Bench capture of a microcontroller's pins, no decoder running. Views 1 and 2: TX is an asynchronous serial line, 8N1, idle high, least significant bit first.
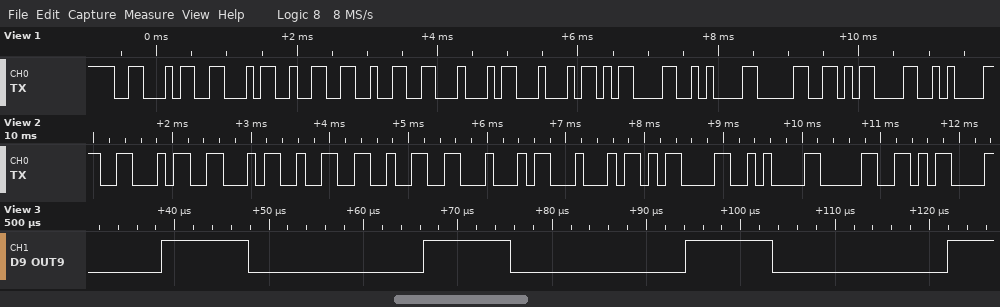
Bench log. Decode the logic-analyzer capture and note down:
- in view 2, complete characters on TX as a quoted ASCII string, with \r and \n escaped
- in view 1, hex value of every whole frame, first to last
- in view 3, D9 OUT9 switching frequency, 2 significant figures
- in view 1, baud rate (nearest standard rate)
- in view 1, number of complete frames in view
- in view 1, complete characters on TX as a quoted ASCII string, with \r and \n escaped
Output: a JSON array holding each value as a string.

["\"FF22DD\\r\\n0\\r\"", "46 46 32 32 44 44 0D 0A 30 0D 0A", "36 kHz", "9600 baud", "11", "\"FF22DD\\r\\n0\\r\\n\""]
